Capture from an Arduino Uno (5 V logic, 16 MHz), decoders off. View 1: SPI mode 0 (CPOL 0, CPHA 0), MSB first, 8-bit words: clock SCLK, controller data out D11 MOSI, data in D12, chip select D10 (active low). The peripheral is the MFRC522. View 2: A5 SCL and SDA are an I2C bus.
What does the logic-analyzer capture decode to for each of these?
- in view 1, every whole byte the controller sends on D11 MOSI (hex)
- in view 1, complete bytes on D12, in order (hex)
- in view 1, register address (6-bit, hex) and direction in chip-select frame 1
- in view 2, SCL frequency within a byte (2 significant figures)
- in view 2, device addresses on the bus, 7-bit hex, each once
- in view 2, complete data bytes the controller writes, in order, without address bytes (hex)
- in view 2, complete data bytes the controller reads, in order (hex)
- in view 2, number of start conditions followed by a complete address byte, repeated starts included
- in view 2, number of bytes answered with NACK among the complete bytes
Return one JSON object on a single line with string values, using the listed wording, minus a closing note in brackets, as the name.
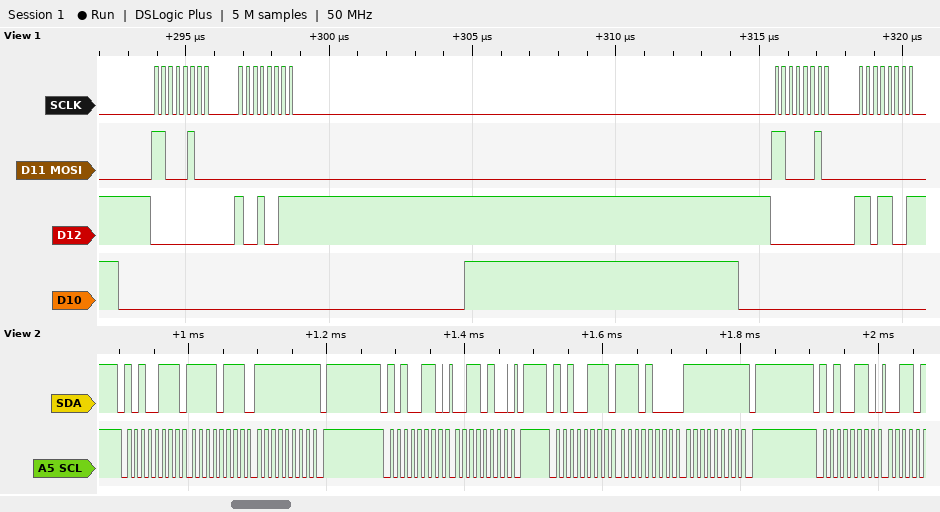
{"in view 1, every whole byte the controller sends on D11 MOSI": "0xC4 0x00 0xC2 0x00", "in view 1, complete bytes on D12, in order": "0x00 0x93 0x00 0xD9", "in view 1, register address (6-bit, hex) and direction in chip-select frame 1": "0x22 read", "in view 2, SCL frequency within a byte": "100 kHz", "in view 2, device addresses on the bus, 7-bit hex, each once": "0x53", "in view 2, complete data bytes the controller writes, in order, without address bytes": "34", "in view 2, complete data bytes the controller reads, in order": "F7 FF E8 FF", "in view 2, number of start conditions followed by a complete address byte, repeated starts included": "4", "in view 2, number of bytes answered with NACK among the complete bytes": "2"}
